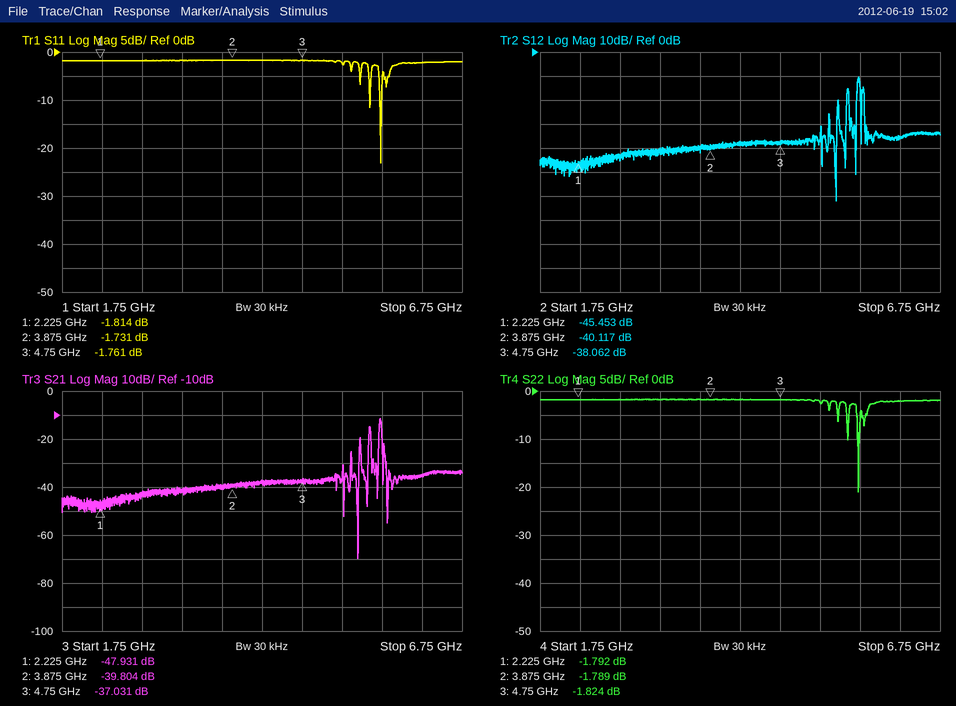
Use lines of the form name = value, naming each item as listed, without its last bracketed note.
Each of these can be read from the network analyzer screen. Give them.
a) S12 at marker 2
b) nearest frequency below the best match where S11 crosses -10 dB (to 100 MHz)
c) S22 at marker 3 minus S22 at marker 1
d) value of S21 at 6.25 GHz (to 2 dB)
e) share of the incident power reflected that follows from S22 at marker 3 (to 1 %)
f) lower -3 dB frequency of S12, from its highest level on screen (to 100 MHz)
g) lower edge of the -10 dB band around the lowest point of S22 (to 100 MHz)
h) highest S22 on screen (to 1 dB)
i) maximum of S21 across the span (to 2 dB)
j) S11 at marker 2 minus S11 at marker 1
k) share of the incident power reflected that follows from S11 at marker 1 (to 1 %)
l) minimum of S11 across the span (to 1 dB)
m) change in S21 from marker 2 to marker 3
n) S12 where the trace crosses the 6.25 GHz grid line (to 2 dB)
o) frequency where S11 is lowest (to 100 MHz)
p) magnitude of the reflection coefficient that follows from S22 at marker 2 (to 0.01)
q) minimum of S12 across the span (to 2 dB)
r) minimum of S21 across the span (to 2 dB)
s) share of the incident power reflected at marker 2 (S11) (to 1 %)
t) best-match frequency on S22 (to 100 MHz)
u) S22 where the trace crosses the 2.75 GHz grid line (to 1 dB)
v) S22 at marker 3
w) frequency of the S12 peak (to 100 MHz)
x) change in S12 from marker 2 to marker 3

S12 at marker 2 = -40.117 dB
nearest frequency below the best match where S11 crosses -10 dB = 5.7 GHz
S22 at marker 3 minus S22 at marker 1 = -0.032 dB
value of S21 at 6.25 GHz = -36 dB
share of the incident power reflected that follows from S22 at marker 3 = 66 %
lower -3 dB frequency of S12, from its highest level on screen = 5.7 GHz
lower edge of the -10 dB band around the lowest point of S22 = 5.7 GHz
highest S22 on screen = -2 dB
maximum of S21 across the span = -12 dB
S11 at marker 2 minus S11 at marker 1 = 0.083 dB
share of the incident power reflected that follows from S11 at marker 1 = 66 %
minimum of S11 across the span = -23 dB
change in S21 from marker 2 to marker 3 = 2.773 dB
S12 where the trace crosses the 6.25 GHz grid line = -36 dB
frequency where S11 is lowest = 5.7 GHz
magnitude of the reflection coefficient that follows from S22 at marker 2 = 0.81
minimum of S12 across the span = -62 dB
minimum of S21 across the span = -70 dB
share of the incident power reflected at marker 2 (S11) = 67 %
best-match frequency on S22 = 5.7 GHz
S22 where the trace crosses the 2.75 GHz grid line = -2 dB
S22 at marker 3 = -1.824 dB
frequency of the S12 peak = 5.7 GHz
change in S12 from marker 2 to marker 3 = 2.055 dB
